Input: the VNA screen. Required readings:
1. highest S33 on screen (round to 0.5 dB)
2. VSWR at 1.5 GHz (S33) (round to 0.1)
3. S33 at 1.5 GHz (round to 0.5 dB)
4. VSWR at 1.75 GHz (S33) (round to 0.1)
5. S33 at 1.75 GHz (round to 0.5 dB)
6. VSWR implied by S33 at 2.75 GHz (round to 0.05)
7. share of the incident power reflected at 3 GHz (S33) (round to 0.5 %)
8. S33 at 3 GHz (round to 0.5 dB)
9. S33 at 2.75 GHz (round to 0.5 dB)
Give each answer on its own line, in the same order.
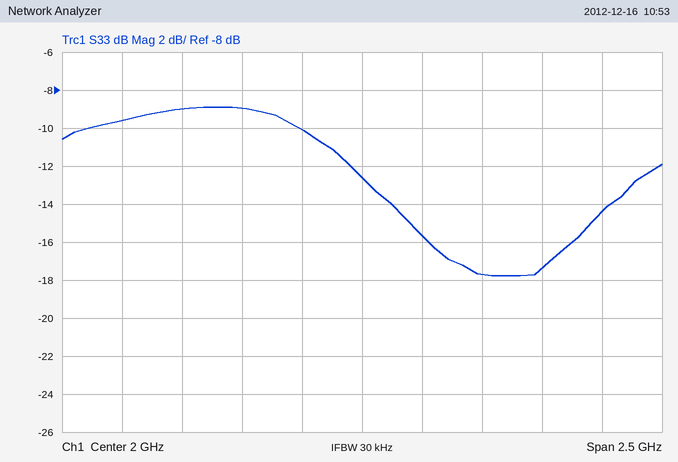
-9.0 dB
2.1
-9.0 dB
1.9
-10.0 dB
1.30
3.5 %
-14.5 dB
-17.5 dB
